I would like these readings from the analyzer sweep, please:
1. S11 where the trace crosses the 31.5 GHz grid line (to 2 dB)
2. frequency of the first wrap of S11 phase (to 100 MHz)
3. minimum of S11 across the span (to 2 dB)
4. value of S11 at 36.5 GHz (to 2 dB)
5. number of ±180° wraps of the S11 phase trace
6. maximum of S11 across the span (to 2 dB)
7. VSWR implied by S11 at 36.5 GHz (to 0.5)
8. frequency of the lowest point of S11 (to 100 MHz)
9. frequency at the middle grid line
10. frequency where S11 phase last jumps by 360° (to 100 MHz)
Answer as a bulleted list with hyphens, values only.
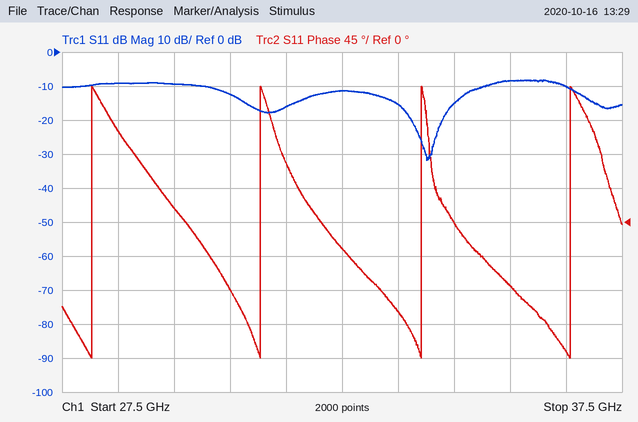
- -16 dB
- 28.0 GHz
- -32 dB
- -10 dB
- 4
- -8 dB
- 2.0
- 34.0 GHz
- 32.5 GHz
- 36.6 GHz
